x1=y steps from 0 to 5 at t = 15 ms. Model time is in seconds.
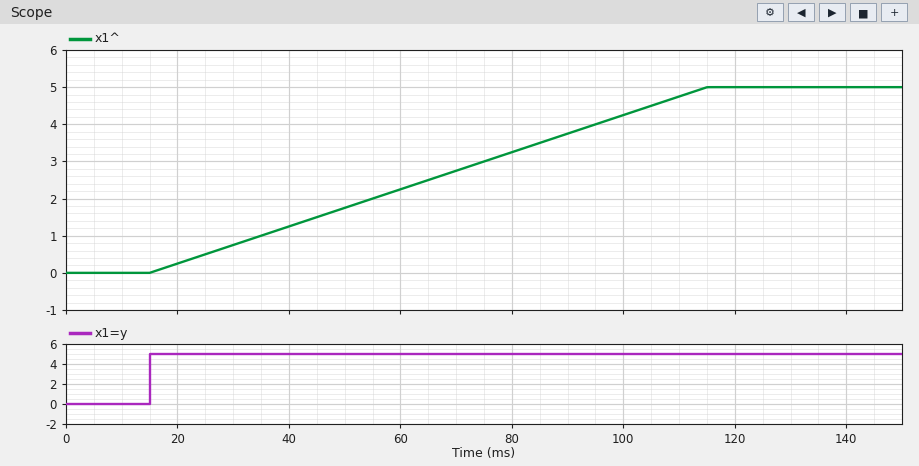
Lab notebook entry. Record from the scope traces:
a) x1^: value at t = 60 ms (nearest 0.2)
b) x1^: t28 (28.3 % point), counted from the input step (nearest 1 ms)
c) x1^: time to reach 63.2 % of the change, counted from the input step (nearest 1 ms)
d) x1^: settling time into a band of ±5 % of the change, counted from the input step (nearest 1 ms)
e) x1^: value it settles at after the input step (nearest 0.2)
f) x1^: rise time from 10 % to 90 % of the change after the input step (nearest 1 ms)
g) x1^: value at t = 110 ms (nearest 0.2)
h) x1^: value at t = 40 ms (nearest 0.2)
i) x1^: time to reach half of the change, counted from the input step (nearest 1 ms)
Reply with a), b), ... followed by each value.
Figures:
a) 2.2
b) 28 ms
c) 63 ms
d) 95 ms
e) 5.0
f) 80 ms
g) 4.8
h) 1.2
i) 50 ms
